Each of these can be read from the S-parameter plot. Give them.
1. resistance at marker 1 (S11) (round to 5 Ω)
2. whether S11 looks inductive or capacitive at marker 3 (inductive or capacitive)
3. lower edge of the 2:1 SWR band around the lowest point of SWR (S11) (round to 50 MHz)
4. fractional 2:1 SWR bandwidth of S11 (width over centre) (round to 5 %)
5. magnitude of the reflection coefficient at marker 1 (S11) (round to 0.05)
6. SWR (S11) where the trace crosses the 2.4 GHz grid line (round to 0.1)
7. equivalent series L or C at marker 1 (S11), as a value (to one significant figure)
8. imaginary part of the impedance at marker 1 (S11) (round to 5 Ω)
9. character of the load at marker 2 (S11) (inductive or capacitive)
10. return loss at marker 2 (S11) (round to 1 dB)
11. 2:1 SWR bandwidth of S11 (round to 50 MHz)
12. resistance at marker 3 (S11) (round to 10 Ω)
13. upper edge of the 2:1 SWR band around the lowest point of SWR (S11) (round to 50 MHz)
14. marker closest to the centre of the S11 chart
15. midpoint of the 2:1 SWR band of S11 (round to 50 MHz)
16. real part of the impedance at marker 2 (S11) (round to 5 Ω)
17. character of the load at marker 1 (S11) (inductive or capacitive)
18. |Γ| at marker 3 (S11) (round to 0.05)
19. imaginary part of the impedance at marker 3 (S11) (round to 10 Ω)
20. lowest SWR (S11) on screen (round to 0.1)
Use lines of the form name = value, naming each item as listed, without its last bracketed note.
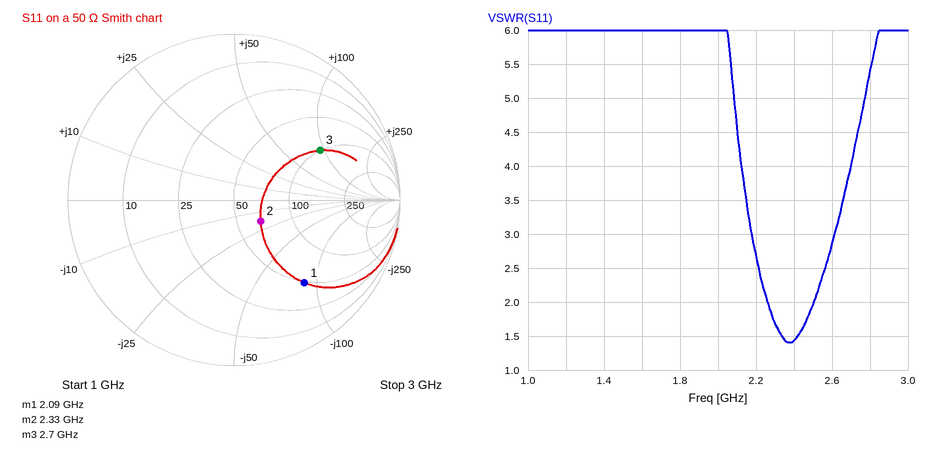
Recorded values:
resistance at marker 1 (S11) = 50 Ω
whether S11 looks inductive or capacitive at marker 3 = inductive
lower edge of the 2:1 SWR band around the lowest point of SWR (S11) = 2.25 GHz
fractional 2:1 SWR bandwidth of S11 (width over centre) = 10 %
magnitude of the reflection coefficient at marker 1 (S11) = 0.65
SWR (S11) where the trace crosses the 2.4 GHz grid line = 1.4
equivalent series L or C at marker 1 (S11), as a value = 900 fF
imaginary part of the impedance at marker 1 (S11) = -85 Ω
character of the load at marker 2 (S11) = capacitive
return loss at marker 2 (S11) = 14 dB
2:1 SWR bandwidth of S11 = 250 MHz
resistance at marker 3 (S11) = 100 Ω
upper edge of the 2:1 SWR band around the lowest point of SWR (S11) = 2.50 GHz
marker closest to the centre of the S11 chart = marker 2
midpoint of the 2:1 SWR band of S11 = 2.40 GHz
real part of the impedance at marker 2 (S11) = 65 Ω
character of the load at marker 1 (S11) = capacitive
|Γ| at marker 3 (S11) = 0.60
imaginary part of the impedance at marker 3 (S11) = +90 Ω
lowest SWR (S11) on screen = 1.4
